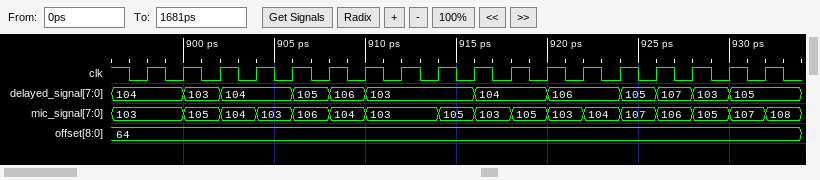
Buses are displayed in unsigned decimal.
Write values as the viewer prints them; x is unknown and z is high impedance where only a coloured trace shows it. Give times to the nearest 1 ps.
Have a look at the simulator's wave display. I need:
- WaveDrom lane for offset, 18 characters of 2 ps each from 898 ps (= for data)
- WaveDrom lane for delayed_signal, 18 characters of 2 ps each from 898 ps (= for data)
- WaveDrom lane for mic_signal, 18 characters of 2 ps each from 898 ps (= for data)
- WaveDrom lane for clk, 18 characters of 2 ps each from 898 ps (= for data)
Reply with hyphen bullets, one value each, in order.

- {name: 'offset', wave: '=.................', data: '64'}
- {name: 'delayed_signal', wave: '===.===..=.=.====.', data: '104 103 104 105 106 103 104 106 105 107 103 105'}
- {name: 'mic_signal', wave: '=======.==========', data: '103 105 104 103 106 104 103 105 103 105 103 104 107 106 105 107 108'}
- {name: 'clk', wave: 'p.................'}
